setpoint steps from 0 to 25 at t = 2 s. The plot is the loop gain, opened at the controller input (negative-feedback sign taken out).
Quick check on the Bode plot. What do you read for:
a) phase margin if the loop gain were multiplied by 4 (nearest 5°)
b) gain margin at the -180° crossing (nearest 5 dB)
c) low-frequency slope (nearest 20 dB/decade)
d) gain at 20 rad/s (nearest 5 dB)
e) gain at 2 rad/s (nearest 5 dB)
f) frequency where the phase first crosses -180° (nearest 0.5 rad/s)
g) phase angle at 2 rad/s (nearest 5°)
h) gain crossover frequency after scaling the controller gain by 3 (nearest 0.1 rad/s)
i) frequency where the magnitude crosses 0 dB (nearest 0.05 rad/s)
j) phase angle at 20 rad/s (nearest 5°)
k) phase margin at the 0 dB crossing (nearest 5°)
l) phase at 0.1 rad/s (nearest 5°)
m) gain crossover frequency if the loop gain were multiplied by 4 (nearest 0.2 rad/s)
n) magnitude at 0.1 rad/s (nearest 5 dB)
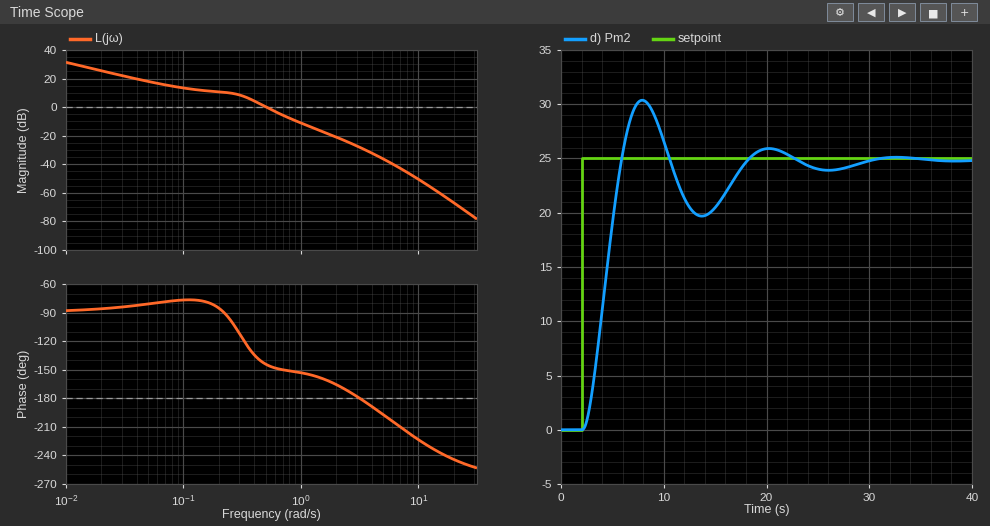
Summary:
25°
30 dB
-20 dB/decade
-65 dB
-20 dB
3.0 rad/s
-165°
0.9 rad/s
0.50 rad/s
-245°
35°
-75°
1.0 rad/s
15 dB
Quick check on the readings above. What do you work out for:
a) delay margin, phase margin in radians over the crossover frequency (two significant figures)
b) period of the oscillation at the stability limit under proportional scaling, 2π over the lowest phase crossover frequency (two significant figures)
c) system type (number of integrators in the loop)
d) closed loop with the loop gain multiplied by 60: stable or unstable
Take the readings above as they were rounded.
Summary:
1.2 s
2.1 s
1
unstable
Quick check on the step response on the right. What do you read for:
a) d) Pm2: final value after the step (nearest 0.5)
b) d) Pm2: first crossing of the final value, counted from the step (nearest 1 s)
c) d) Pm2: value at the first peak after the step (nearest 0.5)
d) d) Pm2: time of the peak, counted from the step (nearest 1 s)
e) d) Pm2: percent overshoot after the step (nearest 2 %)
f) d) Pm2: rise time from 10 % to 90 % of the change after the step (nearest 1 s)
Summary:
25.0
4 s
30.5
6 s
22 %
3 s
